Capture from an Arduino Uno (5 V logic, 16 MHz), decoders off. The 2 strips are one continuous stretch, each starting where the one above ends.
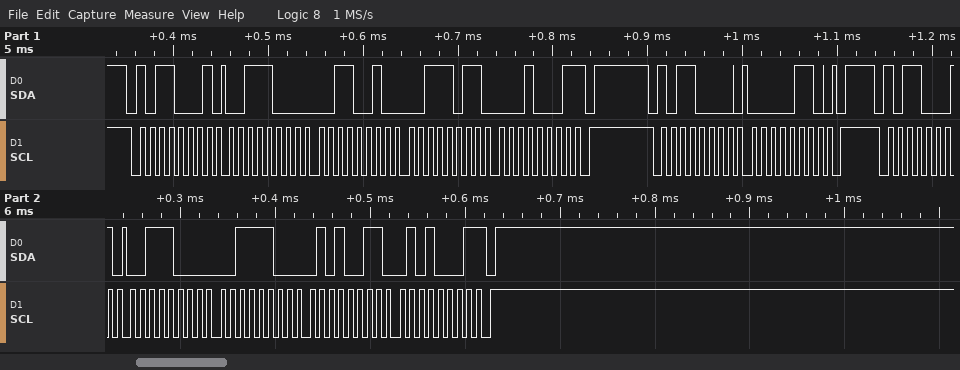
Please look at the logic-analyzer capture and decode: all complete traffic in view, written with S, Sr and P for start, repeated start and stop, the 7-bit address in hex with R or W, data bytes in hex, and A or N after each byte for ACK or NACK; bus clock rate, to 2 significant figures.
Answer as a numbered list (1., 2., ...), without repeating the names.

1. S 58R A 38 A 32 A 3B A 11 N P S 58W A 06 A P S 58R A 38 A 3C A 53 A 51 N P
2. 100 kHz
